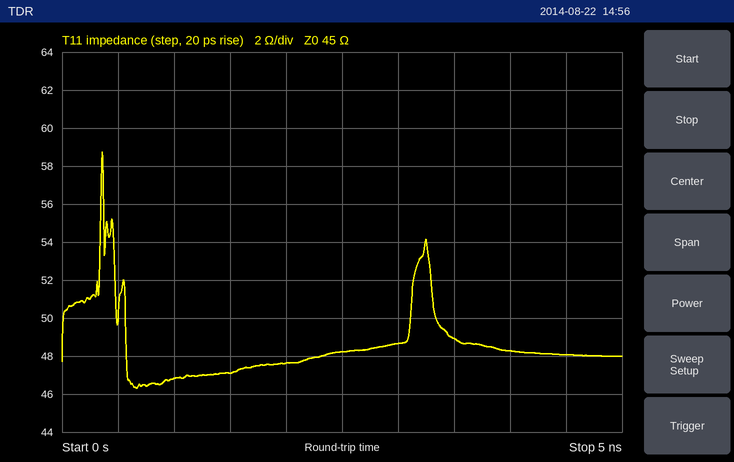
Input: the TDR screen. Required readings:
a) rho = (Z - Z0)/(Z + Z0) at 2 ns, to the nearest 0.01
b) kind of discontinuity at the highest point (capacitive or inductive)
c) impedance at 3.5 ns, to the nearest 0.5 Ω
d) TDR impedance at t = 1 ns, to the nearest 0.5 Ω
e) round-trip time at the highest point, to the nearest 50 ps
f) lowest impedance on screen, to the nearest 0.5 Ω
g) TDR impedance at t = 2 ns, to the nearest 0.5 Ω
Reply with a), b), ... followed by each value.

a) +0.03
b) inductive
c) 49.0 Ω
d) 47.0 Ω
e) 350 ps
f) 46.5 Ω
g) 47.5 Ω
